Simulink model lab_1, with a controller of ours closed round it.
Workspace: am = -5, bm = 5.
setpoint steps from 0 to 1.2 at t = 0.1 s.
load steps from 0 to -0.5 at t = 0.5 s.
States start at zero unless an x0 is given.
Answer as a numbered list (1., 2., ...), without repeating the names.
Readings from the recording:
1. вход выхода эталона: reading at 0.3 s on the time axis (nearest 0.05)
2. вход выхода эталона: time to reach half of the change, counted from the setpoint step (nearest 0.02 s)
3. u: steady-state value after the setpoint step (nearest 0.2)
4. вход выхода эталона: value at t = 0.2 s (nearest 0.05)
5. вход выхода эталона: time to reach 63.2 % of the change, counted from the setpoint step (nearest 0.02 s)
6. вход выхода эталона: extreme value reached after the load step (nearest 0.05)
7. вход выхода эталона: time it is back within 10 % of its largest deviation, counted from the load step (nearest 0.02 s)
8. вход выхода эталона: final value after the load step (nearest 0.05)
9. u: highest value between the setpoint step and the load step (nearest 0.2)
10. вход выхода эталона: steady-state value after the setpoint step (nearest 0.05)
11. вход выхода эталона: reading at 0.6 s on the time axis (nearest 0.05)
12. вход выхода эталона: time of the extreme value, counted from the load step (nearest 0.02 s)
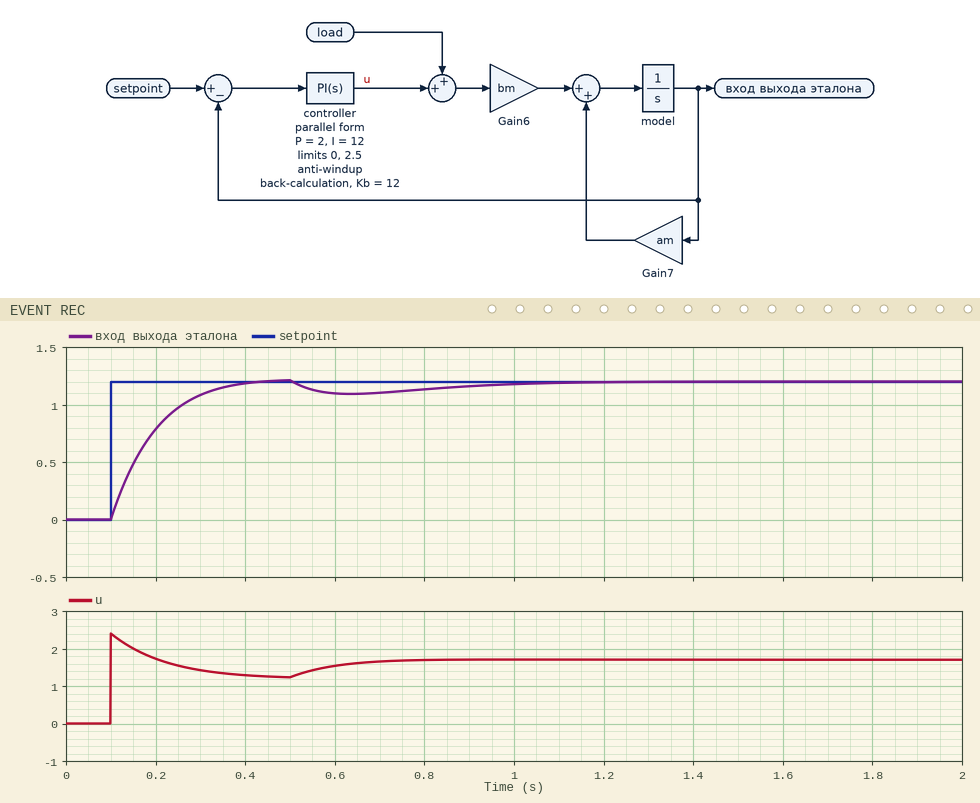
1. 1.10
2. 0.06 s
3. 1.2
4. 0.80
5. 0.10 s
6. 1.10
7. 0.60 s
8. 1.20
9. 2.4
10. 1.20
11. 1.10
12. 0.14 s
